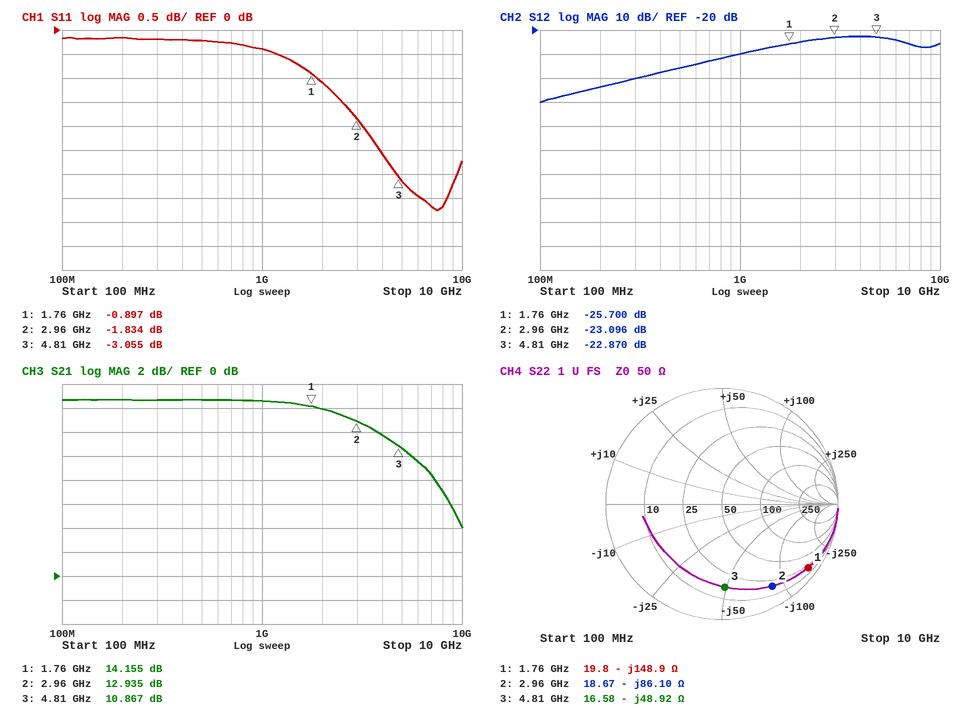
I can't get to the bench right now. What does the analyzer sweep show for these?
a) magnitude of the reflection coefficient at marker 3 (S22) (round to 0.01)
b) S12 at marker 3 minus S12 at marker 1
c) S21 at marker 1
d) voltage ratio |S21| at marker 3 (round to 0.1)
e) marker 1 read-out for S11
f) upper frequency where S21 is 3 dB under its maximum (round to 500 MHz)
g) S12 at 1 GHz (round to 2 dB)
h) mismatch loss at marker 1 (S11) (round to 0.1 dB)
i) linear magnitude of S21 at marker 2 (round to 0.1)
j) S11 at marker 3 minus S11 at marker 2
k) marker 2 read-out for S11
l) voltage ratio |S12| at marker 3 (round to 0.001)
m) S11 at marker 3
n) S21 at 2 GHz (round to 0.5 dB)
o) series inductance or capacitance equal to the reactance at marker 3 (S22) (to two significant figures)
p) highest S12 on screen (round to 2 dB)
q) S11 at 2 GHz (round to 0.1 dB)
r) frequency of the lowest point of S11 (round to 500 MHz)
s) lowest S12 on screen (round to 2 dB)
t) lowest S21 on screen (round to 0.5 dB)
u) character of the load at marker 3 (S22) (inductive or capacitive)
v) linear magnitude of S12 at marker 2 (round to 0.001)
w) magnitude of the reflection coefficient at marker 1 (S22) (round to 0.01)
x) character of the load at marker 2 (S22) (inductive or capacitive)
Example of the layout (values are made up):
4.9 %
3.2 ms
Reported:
0.72
2.830 dB
14.155 dB
3.5
-0.897 dB
4.0 GHz
-30 dB
7.3 dB
4.4
-1.221 dB
-1.834 dB
0.072
-3.055 dB
14.0 dB
680 fF
-22 dB
-1.1 dB
7.5 GHz
-50 dB
4.0 dB
capacitive
0.070
0.92
capacitive
